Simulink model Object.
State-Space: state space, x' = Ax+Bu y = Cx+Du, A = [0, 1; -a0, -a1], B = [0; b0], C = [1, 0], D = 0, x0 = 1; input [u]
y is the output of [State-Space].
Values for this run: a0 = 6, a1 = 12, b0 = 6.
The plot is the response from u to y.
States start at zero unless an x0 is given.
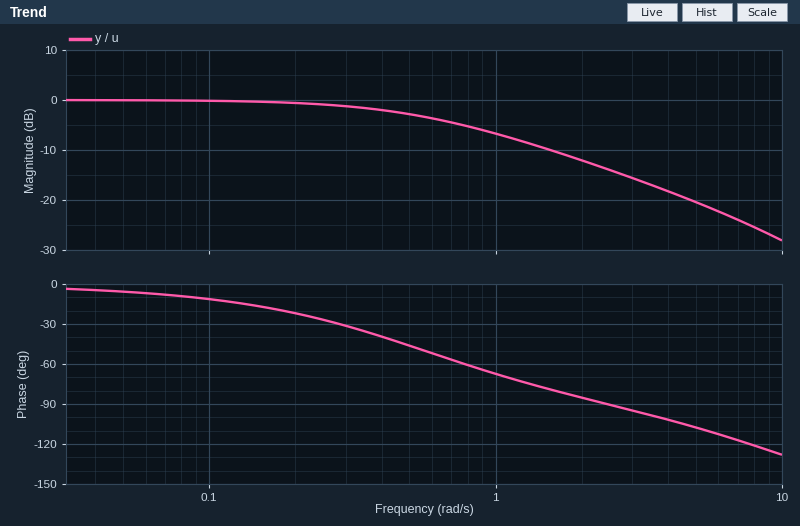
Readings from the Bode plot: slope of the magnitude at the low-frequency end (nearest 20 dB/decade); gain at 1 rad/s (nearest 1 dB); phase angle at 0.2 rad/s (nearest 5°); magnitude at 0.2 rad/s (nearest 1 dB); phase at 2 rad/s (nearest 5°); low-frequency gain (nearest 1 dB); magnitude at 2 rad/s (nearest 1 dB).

0 dB/decade
-7 dB
-20°
-1 dB
-85°
0 dB
-12 dB
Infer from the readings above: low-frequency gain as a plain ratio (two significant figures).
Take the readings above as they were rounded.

1.0
